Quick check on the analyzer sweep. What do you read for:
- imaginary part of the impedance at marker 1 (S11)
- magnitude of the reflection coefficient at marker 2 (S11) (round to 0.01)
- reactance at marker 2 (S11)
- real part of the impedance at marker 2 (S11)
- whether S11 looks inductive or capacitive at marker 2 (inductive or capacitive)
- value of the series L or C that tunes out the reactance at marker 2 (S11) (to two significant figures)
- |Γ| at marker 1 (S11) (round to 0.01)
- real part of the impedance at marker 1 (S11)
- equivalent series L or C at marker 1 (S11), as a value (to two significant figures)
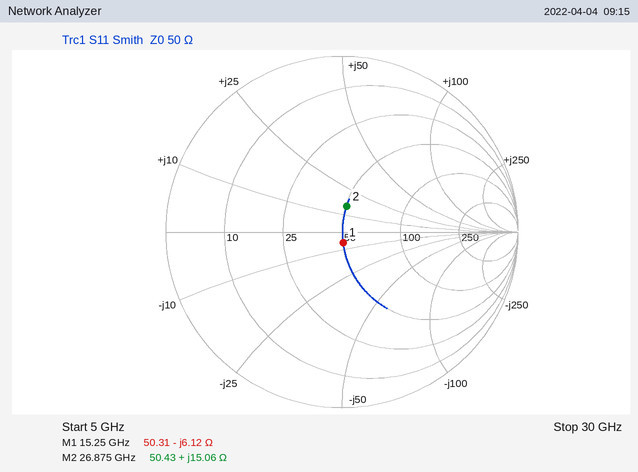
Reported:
-6.12 Ω
0.15
+15.06 Ω
50.43 Ω
inductive
390 fF
0.06
50.31 Ω
1.7 pF
